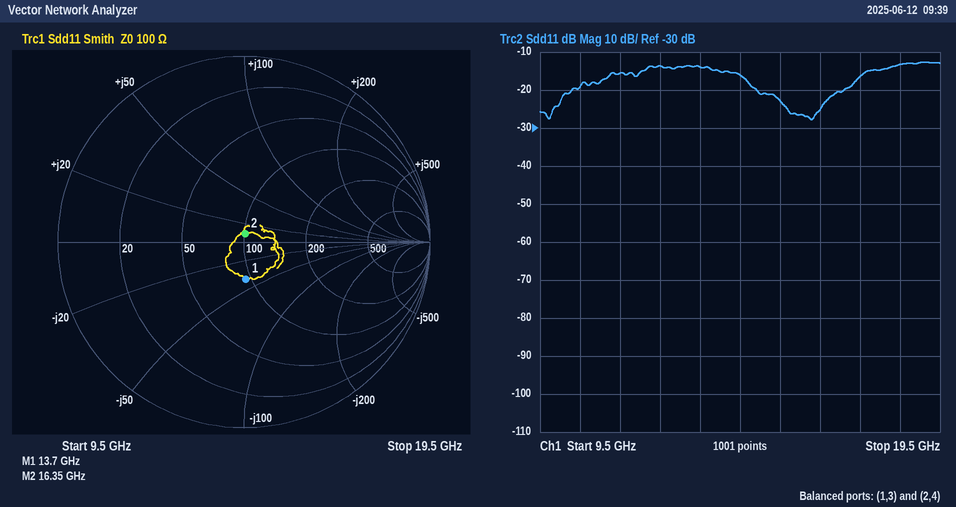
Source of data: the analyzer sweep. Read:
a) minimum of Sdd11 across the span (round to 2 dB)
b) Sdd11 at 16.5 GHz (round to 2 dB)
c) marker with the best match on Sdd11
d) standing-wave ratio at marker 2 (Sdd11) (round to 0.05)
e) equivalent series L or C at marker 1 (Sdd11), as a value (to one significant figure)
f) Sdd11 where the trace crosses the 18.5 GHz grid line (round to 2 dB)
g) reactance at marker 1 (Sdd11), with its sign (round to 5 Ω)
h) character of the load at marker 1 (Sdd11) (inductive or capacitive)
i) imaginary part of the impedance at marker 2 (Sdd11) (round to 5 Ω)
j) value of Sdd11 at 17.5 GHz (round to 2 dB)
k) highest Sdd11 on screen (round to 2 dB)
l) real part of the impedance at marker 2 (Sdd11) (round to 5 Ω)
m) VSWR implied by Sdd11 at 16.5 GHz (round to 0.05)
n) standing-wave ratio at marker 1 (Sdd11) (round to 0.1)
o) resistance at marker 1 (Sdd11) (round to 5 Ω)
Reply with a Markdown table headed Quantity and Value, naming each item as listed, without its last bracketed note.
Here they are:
| Quantity | Value |
|---|---|
| minimum of Sdd11 across the span | -28 dB |
| Sdd11 at 16.5 GHz | -26 dB |
| marker with the best match on Sdd11 | marker 2 |
| standing-wave ratio at marker 2 (Sdd11) | 1.10 |
| equivalent series L or C at marker 1 (Sdd11), as a value | 300 fF |
| Sdd11 where the trace crosses the 18.5 GHz grid line | -14 dB |
| reactance at marker 1 (Sdd11), with its sign | -40 Ω |
| character of the load at marker 1 (Sdd11) | capacitive |
| imaginary part of the impedance at marker 2 (Sdd11) | +10 Ω |
| value of Sdd11 at 17.5 GHz | -16 dB |
| highest Sdd11 on screen | -12 dB |
| real part of the impedance at marker 2 (Sdd11) | 100 Ω |
| VSWR implied by Sdd11 at 16.5 GHz | 1.10 |
| standing-wave ratio at marker 1 (Sdd11) | 1.5 |
| resistance at marker 1 (Sdd11) | 95 Ω |
